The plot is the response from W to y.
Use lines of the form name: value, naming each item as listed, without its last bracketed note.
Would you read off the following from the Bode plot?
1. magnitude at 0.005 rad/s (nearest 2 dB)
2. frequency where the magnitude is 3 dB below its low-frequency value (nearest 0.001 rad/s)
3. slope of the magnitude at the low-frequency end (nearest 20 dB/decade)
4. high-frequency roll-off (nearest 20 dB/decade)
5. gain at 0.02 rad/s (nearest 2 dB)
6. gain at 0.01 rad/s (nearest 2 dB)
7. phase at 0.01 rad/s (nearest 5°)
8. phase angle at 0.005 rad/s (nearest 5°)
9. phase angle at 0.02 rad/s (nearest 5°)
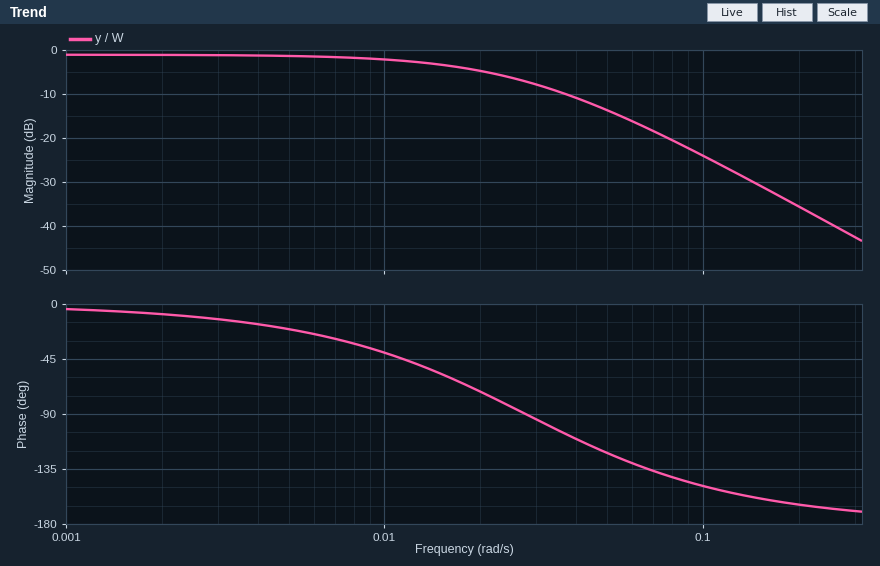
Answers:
magnitude at 0.005 rad/s: -2 dB
frequency where the magnitude is 3 dB below its low-frequency value: 0.018 rad/s
slope of the magnitude at the low-frequency end: 0 dB/decade
high-frequency roll-off: -40 dB/decade
gain at 0.02 rad/s: -4 dB
gain at 0.01 rad/s: -2 dB
phase at 0.01 rad/s: -40°
phase angle at 0.005 rad/s: -20°
phase angle at 0.02 rad/s: -70°
